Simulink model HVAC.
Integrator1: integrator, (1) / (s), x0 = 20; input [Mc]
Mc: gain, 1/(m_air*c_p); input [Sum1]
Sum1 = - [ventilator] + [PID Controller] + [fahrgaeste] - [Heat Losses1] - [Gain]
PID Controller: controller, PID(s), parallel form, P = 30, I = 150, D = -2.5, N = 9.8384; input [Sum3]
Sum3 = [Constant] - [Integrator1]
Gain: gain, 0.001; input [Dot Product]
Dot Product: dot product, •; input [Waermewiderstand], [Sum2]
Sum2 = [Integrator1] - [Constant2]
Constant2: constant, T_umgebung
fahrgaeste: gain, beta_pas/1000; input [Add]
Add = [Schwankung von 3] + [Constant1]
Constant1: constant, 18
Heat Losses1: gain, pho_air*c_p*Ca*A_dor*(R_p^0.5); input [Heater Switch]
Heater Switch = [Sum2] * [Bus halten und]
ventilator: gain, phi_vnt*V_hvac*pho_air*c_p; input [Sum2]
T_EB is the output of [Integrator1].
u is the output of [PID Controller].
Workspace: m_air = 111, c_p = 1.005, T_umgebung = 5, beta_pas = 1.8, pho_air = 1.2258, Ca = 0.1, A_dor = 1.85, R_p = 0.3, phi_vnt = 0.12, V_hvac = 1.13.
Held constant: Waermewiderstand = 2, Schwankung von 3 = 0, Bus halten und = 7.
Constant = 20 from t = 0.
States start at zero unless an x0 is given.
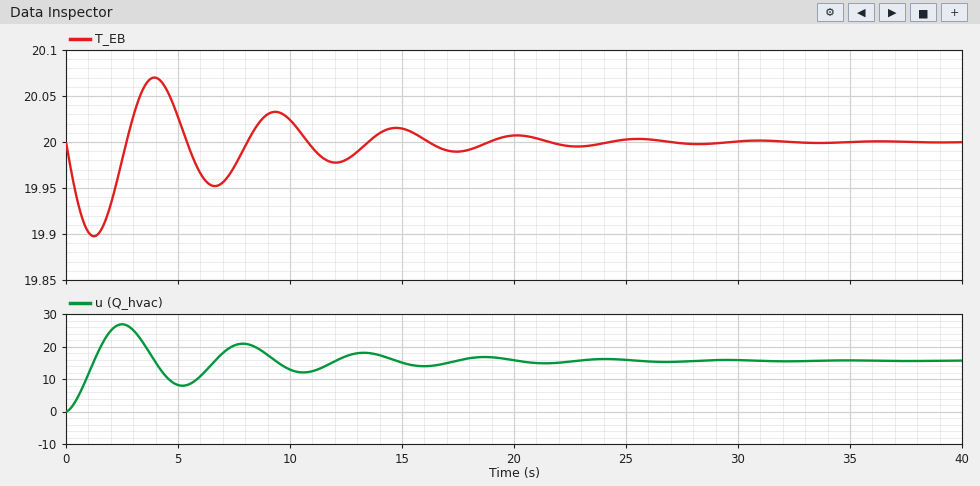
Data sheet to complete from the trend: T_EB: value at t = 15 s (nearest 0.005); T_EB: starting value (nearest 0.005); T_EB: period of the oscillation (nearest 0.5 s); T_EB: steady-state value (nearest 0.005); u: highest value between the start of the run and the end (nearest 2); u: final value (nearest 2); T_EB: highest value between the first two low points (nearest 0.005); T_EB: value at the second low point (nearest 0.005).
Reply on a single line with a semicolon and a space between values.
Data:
20.015; 20.000; 5.5 s; 20.000; 26; 16; 20.070; 19.950
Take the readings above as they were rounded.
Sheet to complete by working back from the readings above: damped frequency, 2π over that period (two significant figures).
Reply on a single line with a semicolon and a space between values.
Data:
1.1 rad/s
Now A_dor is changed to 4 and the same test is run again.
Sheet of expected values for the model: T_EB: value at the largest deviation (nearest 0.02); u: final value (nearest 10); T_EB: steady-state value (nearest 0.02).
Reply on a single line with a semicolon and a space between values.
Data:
19.80; 30; 20.00
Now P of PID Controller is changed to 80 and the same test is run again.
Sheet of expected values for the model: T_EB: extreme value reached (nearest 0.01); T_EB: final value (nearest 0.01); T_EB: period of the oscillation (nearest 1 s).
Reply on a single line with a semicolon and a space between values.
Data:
19.92; 20.00; 6 s
